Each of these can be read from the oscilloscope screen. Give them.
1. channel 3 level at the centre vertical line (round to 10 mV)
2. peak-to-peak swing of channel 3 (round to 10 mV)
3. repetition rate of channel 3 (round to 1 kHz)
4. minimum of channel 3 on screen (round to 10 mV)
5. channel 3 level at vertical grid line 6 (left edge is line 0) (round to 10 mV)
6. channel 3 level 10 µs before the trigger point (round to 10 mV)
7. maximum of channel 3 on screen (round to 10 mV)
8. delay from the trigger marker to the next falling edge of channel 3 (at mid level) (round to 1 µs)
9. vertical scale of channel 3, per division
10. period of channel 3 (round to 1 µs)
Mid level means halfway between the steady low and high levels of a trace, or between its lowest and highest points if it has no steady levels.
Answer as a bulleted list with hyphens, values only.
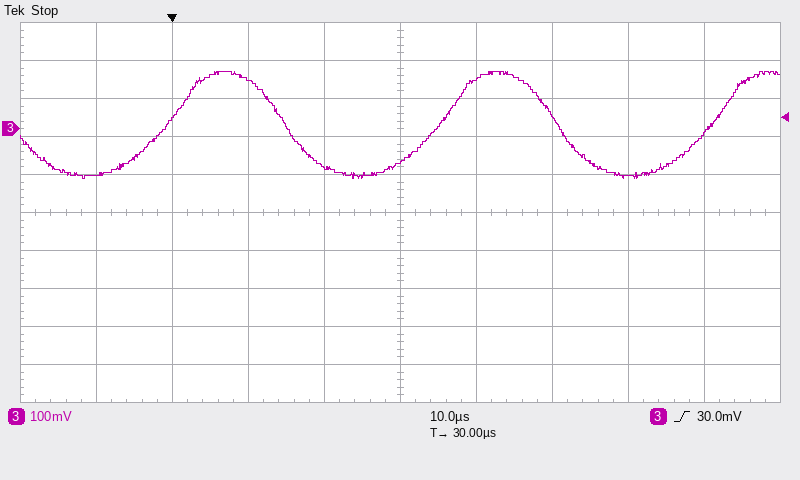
- -90 mV
- 280 mV
- 28 kHz
- -130 mV
- 130 mV
- -120 mV
- 150 mV
- 15 µs
- 100 mV
- 36 µs
